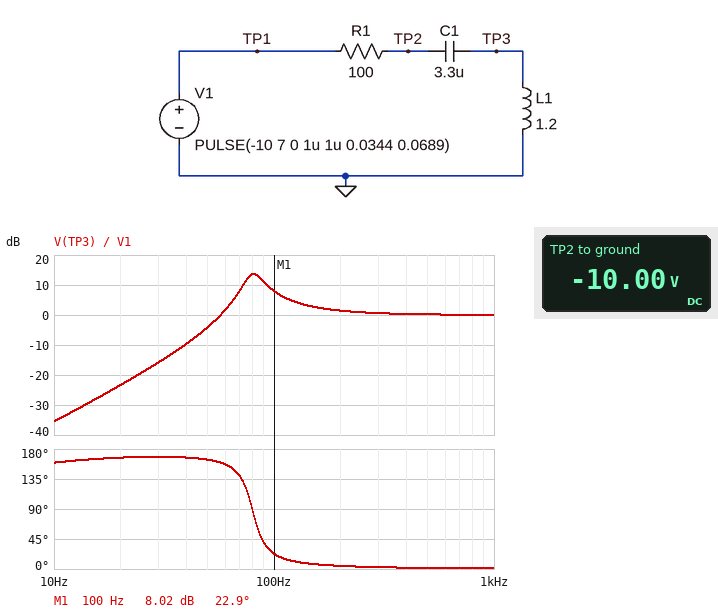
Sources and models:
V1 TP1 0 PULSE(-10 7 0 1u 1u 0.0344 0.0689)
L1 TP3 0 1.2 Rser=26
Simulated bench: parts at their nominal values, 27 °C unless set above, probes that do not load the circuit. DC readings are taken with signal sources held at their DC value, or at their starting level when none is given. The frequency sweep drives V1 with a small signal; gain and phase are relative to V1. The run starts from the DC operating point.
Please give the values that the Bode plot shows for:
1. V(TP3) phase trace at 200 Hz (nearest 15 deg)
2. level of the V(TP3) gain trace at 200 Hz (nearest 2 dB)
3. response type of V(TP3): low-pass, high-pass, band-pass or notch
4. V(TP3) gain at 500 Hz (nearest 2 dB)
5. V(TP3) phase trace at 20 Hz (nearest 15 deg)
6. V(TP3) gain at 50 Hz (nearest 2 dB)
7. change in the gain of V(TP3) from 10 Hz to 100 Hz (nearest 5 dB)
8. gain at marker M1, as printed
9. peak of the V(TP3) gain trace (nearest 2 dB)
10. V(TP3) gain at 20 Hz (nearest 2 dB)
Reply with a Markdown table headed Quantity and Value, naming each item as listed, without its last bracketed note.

| Quantity | Value |
|---|---|
| V(TP3) phase trace at 200 Hz | 0 deg |
| level of the V(TP3) gain trace at 200 Hz | 2 dB |
| response type of V(TP3): low-pass, high-pass, band-pass or notch | high-pass |
| V(TP3) gain at 500 Hz | 0 dB |
| V(TP3) phase trace at 20 Hz | 165 deg |
| V(TP3) gain at 50 Hz | -4 dB |
| change in the gain of V(TP3) from 10 Hz to 100 Hz | 45 dB |
| gain at marker M1, as printed | 8.02 dB |
| peak of the V(TP3) gain trace | 14 dB |
| V(TP3) gain at 20 Hz | -24 dB |
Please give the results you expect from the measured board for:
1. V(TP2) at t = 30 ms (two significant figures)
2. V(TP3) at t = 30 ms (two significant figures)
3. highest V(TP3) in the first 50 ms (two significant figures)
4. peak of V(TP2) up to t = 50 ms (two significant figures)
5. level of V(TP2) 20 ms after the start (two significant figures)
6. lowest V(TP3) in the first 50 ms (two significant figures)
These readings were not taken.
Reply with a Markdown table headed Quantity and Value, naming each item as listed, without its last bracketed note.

| Quantity | Value |
|---|---|
| V(TP2) at t = 30 ms | 6.6 V |
| V(TP3) at t = 30 ms | -2.8 V |
| highest V(TP3) in the first 50 ms | 17 V |
| peak of V(TP2) up to t = 50 ms | 8.7 V |
| level of V(TP2) 20 ms after the start | 7.5 V |
| lowest V(TP3) in the first 50 ms | -17 V |
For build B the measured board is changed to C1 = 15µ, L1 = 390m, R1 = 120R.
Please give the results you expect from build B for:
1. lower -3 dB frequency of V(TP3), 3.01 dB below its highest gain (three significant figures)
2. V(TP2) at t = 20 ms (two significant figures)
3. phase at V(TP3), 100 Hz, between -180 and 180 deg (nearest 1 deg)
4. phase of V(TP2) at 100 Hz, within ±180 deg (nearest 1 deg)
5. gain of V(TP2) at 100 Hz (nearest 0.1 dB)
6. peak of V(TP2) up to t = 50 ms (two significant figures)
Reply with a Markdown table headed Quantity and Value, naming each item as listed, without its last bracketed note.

| Quantity | Value |
|---|---|
| lower -3 dB frequency of V(TP3), 3.01 dB below its highest gain | 55.3 Hz |
| V(TP2) at t = 20 ms | 6.7 V |
| phase at V(TP3), 100 Hz, between -180 and 180 deg | 40 deg |
| phase of V(TP2) at 100 Hz, within ±180 deg | 36 deg |
| gain of V(TP2) at 100 Hz | -3.1 dB |
| peak of V(TP2) up to t = 50 ms | 8.5 V |
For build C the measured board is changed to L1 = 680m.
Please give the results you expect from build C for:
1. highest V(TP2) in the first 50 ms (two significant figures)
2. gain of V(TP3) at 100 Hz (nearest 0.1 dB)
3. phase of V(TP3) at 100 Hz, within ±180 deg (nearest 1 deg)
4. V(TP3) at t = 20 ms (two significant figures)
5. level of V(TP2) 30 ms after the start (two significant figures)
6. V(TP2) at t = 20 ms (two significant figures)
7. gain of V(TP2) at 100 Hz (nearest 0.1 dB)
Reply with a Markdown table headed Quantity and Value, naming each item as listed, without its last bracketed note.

| Quantity | Value |
|---|---|
| highest V(TP2) in the first 50 ms | 9.0 V |
| gain of V(TP3) at 100 Hz | 9.9 dB |
| phase of V(TP3) at 100 Hz, within ±180 deg | 110 deg |
| V(TP3) at t = 20 ms | 2.0 V |
| level of V(TP2) 30 ms after the start | 6.8 V |
| V(TP2) at t = 20 ms | 6.6 V |
| gain of V(TP2) at 100 Hz | -7.1 dB |
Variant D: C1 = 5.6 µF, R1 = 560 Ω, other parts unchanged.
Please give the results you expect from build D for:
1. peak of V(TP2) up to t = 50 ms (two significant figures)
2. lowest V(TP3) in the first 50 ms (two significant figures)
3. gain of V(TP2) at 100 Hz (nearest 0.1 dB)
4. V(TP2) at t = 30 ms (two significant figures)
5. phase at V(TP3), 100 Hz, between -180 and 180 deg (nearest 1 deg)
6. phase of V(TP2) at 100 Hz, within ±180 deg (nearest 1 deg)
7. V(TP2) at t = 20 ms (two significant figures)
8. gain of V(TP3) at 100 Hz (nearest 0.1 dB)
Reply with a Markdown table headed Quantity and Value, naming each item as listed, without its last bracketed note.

| Quantity | Value |
|---|---|
| peak of V(TP2) up to t = 50 ms | 7.8 V |
| lowest V(TP3) in the first 50 ms | -17 V |
| gain of V(TP2) at 100 Hz | -4.1 dB |
| V(TP2) at t = 30 ms | 7.0 V |
| phase at V(TP3), 100 Hz, between -180 and 180 deg | 49 deg |
| phase of V(TP2) at 100 Hz, within ±180 deg | 48 deg |
| V(TP2) at t = 20 ms | 7.1 V |
| gain of V(TP3) at 100 Hz | 0 dB |
